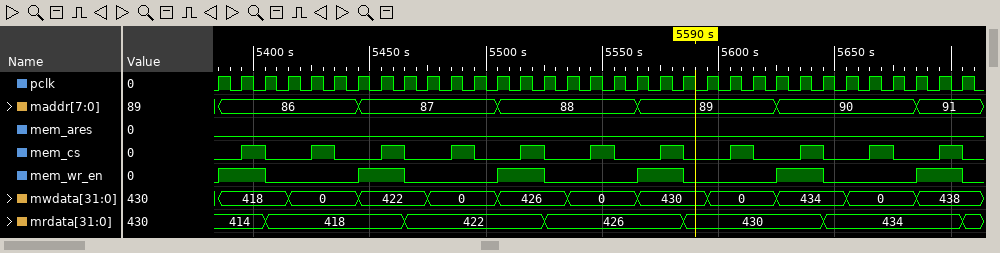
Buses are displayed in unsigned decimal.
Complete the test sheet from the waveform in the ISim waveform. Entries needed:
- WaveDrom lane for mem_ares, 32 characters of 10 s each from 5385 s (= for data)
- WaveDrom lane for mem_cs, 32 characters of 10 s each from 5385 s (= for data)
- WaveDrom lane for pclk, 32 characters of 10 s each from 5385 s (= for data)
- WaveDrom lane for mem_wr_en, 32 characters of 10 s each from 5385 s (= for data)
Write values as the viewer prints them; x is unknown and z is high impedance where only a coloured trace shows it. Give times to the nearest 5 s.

{name: 'mem_ares', wave: '0...............................'}
{name: 'mem_cs', wave: '010.10.10.10.10.10.10.10.10.10.1'}
{name: 'pclk', wave: 'p...............................'}
{name: 'mem_wr_en', wave: '1.0...1.0...1.0...1.0...1.0...1.'}
